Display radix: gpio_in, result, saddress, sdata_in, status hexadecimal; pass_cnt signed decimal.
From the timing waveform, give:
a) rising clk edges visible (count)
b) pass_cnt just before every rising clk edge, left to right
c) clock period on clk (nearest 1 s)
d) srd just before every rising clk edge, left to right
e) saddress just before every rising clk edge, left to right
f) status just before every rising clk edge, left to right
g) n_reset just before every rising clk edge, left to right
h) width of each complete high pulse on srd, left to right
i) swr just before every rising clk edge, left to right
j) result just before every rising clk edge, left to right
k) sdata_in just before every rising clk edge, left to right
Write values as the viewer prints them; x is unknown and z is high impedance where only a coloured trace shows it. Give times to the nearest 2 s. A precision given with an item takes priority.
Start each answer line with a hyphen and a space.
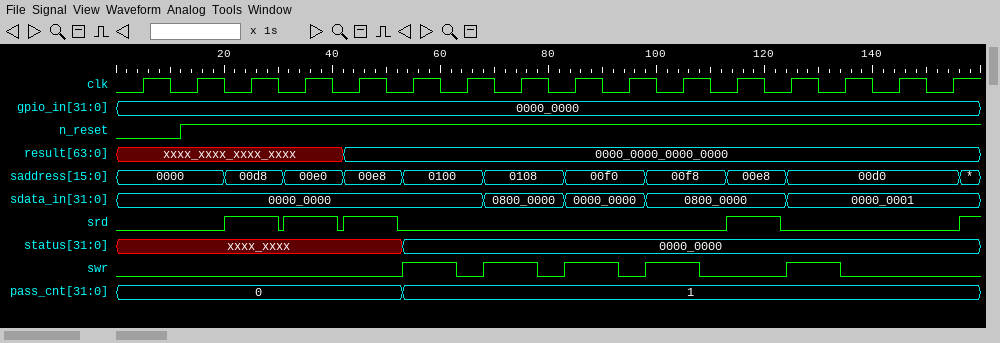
- 16
- 0, 0, 0, 0, 0, 1, 1, 1, 1, 1, 1, 1, 1, 1, 1, 1
- 10 s
- 0 0 1 1 1 0 0 0 0 0 0 1 0 0 0 0
- 0000, 0000, 00d8, 00e0, 00e8, 0100, 0100, 0108, 00f0, 00f0, 00f8, 00e8, 00d0, 00d0, 00d0, 00d0
- xxxx_xxxx, xxxx_xxxx, xxxx_xxxx, xxxx_xxxx, xxxx_xxxx, 0000_0000, 0000_0000, 0000_0000, 0000_0000, 0000_0000, 0000_0000, 0000_0000, 0000_0000, 0000_0000, 0000_0000, 0000_0000
- 0 1 1 1 1 1 1 1 1 1 1 1 1 1 1 1
- 10 s, 10 s, 10 s, 10 s
- 0 0 0 0 0 1 0 1 1 0 1 0 1 0 0 0
- xxxx_xxxx_xxxx_xxxx, xxxx_xxxx_xxxx_xxxx, xxxx_xxxx_xxxx_xxxx, xxxx_xxxx_xxxx_xxxx, 0000_0000_0000_0000, 0000_0000_0000_0000, 0000_0000_0000_0000, 0000_0000_0000_0000, 0000_0000_0000_0000, 0000_0000_0000_0000, 0000_0000_0000_0000, 0000_0000_0000_0000, 0000_0000_0000_0000, 0000_0000_0000_0000, 0000_0000_0000_0000, 0000_0000_0000_0000
- 0000_0000, 0000_0000, 0000_0000, 0000_0000, 0000_0000, 0000_0000, 0000_0000, 0800_0000, 0000_0000, 0000_0000, 0800_0000, 0800_0000, 0000_0001, 0000_0001, 0000_0001, 0000_0001
